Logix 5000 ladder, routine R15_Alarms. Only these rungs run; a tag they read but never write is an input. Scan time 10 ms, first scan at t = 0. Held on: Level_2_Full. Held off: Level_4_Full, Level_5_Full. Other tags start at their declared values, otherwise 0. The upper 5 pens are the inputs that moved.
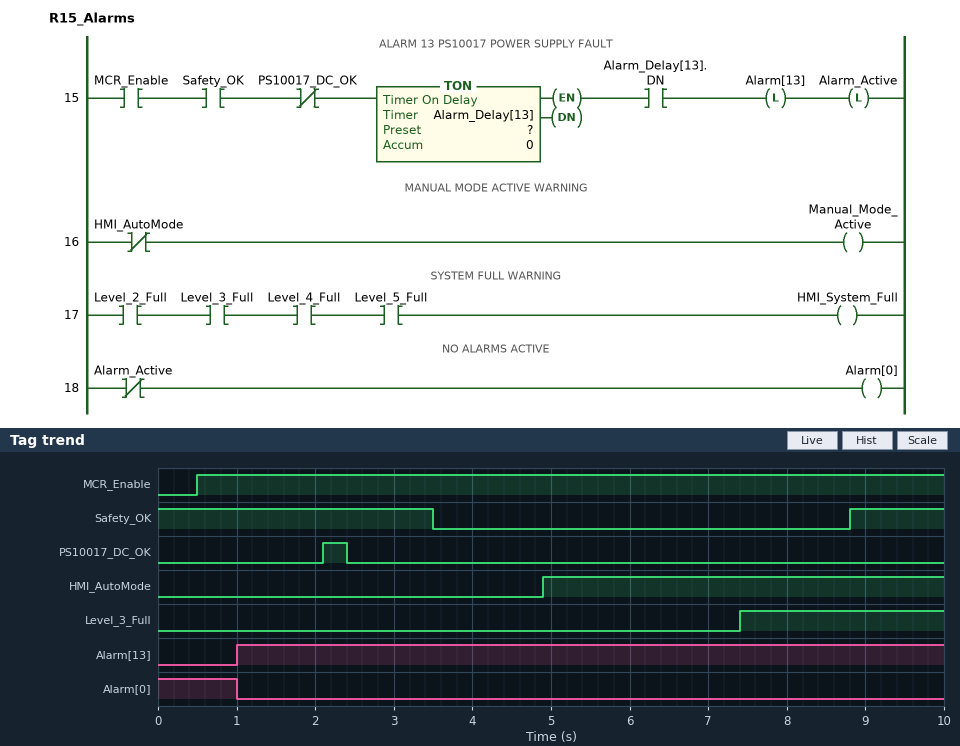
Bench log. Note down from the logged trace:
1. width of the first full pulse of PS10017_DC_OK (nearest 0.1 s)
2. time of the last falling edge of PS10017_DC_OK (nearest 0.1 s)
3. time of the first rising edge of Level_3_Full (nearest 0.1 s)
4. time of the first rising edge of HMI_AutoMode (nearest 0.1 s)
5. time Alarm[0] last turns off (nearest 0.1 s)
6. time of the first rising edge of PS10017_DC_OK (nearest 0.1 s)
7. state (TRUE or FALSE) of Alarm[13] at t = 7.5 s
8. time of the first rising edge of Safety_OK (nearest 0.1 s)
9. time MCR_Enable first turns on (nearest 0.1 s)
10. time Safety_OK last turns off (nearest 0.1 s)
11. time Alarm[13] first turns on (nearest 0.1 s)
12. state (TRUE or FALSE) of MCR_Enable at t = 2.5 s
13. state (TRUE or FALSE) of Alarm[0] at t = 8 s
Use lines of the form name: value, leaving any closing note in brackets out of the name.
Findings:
width of the first full pulse of PS10017_DC_OK: 0.3 s
time of the last falling edge of PS10017_DC_OK: 2.4 s
time of the first rising edge of Level_3_Full: 7.4 s
time of the first rising edge of HMI_AutoMode: 4.9 s
time Alarm[0] last turns off: 1.0 s
time of the first rising edge of PS10017_DC_OK: 2.1 s
state (TRUE or FALSE) of Alarm[13] at t = 7.5 s: TRUE
time of the first rising edge of Safety_OK: 8.8 s
time MCR_Enable first turns on: 0.5 s
time Safety_OK last turns off: 3.5 s
time Alarm[13] first turns on: 1.0 s
state (TRUE or FALSE) of MCR_Enable at t = 2.5 s: TRUE
state (TRUE or FALSE) of Alarm[0] at t = 8 s: FALSE
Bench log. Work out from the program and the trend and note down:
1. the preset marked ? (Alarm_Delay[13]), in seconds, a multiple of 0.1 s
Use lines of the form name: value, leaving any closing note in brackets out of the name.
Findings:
the preset marked ? (Alarm_Delay[13]), in seconds, a multiple of 0.1 s: 0.5 s
